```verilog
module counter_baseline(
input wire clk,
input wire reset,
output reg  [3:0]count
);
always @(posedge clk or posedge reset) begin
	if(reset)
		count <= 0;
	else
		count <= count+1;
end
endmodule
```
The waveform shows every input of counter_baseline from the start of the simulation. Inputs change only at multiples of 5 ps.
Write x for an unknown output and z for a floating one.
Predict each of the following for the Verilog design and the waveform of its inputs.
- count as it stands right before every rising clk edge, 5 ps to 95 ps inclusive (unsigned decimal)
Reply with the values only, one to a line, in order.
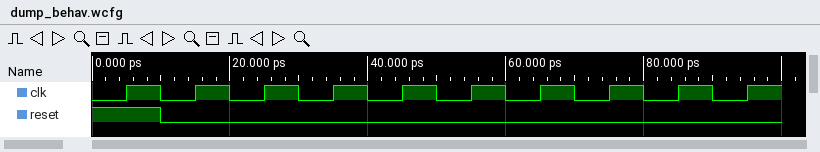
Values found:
0, 0, 1, 2, 3, 4, 5, 6, 7, 8
